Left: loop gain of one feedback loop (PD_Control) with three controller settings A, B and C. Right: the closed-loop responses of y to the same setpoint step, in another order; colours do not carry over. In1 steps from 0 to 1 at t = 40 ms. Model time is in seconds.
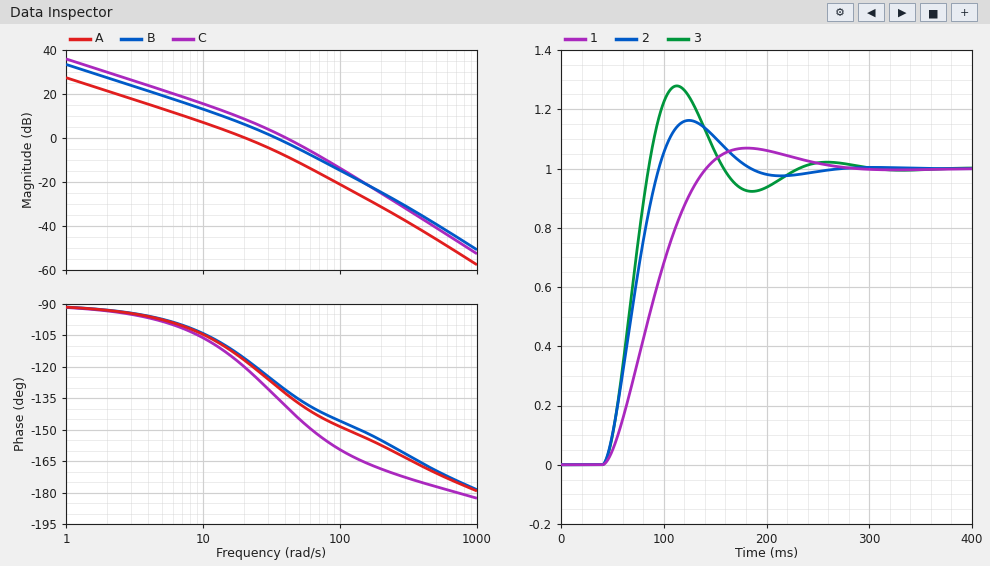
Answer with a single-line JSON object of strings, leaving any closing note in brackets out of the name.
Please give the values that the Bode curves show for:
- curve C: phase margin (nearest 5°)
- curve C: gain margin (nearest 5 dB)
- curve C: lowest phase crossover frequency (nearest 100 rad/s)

{"curve C: phase margin": "40°", "curve C: gain margin": "45 dB", "curve C: lowest phase crossover frequency": "700 rad/s"}
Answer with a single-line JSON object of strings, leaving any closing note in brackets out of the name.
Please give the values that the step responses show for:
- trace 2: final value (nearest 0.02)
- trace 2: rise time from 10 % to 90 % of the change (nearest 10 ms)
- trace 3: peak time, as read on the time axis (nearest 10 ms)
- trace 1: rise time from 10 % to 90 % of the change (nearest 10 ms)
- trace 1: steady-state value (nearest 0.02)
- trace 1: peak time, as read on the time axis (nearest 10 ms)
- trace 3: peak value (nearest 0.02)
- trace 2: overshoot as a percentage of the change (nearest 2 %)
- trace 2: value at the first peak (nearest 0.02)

{"trace 2: final value": "1.00", "trace 2: rise time from 10 % to 90 % of the change": "40 ms", "trace 3: peak time, as read on the time axis": "110 ms", "trace 1: rise time from 10 % to 90 % of the change": "70 ms", "trace 1: steady-state value": "1.00", "trace 1: peak time, as read on the time axis": "180 ms", "trace 3: peak value": "1.28", "trace 2: overshoot as a percentage of the change": "16 %", "trace 2: value at the first peak": "1.16"}
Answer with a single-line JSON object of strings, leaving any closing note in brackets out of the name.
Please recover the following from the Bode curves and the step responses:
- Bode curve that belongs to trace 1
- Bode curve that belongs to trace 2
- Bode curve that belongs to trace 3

{"Bode curve that belongs to trace 1": "A", "Bode curve that belongs to trace 2": "B", "Bode curve that belongs to trace 3": "C"}
